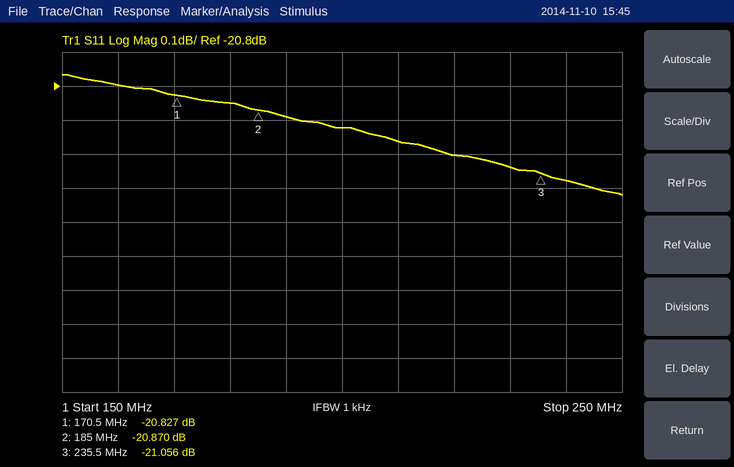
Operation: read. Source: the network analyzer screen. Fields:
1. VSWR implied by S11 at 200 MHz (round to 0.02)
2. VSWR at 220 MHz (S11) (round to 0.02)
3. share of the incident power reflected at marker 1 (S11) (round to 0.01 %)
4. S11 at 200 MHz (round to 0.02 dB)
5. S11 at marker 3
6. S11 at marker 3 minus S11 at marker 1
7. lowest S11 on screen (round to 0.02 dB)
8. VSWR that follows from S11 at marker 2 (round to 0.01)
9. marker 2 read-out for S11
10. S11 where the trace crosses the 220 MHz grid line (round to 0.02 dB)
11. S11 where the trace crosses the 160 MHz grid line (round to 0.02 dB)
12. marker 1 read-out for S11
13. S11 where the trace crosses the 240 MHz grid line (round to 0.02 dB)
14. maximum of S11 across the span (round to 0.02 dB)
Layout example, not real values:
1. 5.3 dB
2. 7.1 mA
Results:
1. 1.20
2. 1.20
3. 0.83 %
4. -20.92 dB
5. -21.056 dB
6. -0.229 dB
7. -21.12 dB
8. 1.20
9. -20.870 dB
10. -21.00 dB
11. -20.80 dB
12. -20.827 dB
13. -21.08 dB
14. -20.76 dB
